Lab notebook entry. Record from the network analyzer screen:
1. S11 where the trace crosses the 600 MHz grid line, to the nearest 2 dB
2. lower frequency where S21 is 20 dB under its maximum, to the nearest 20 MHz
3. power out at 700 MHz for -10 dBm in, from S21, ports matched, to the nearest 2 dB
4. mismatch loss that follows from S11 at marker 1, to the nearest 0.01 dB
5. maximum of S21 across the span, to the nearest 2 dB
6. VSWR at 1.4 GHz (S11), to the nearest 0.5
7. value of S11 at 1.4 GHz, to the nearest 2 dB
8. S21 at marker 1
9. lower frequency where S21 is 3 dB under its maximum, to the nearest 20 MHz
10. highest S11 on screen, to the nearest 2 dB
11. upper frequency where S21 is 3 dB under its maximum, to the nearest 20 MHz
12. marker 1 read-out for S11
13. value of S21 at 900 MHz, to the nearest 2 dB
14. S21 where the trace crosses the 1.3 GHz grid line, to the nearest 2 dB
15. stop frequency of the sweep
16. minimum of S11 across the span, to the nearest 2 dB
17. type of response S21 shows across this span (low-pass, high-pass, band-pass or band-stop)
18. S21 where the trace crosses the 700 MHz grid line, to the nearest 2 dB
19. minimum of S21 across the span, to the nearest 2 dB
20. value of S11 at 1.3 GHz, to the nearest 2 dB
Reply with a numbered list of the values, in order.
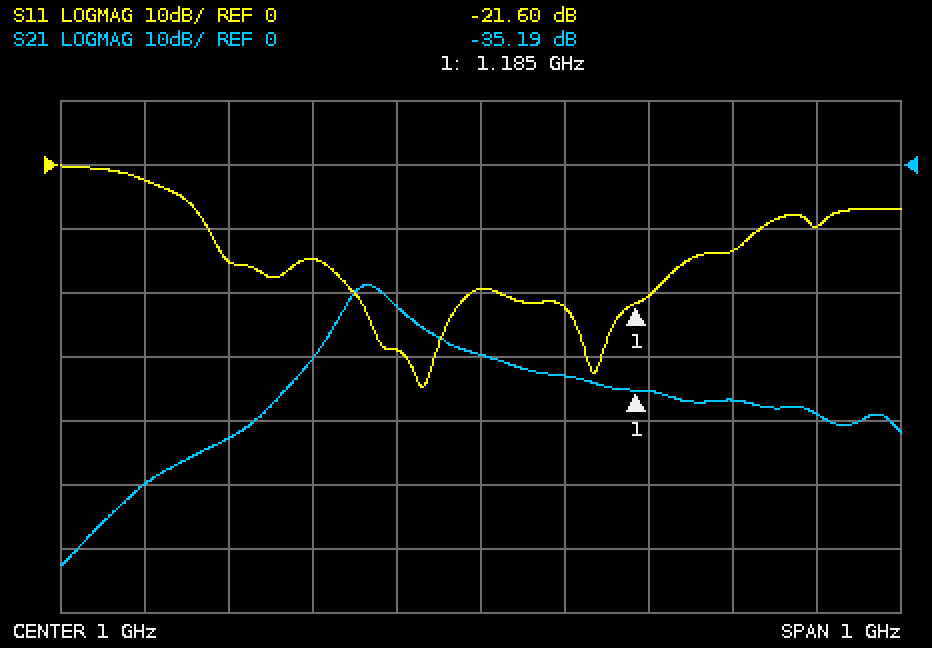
1. -2 dB
2. 740 MHz
3. -52 dBm
4. 0.03 dB
5. -18 dB
6. 2.0
7. -10 dB
8. -35.19 dB
9. 840 MHz
10. 0 dB
11. 900 MHz
12. -21.60 dB
13. -22 dB
14. -36 dB
15. 1.5 GHz
16. -34 dB
17. band-pass
18. -42 dB
19. -62 dB
20. -14 dB
